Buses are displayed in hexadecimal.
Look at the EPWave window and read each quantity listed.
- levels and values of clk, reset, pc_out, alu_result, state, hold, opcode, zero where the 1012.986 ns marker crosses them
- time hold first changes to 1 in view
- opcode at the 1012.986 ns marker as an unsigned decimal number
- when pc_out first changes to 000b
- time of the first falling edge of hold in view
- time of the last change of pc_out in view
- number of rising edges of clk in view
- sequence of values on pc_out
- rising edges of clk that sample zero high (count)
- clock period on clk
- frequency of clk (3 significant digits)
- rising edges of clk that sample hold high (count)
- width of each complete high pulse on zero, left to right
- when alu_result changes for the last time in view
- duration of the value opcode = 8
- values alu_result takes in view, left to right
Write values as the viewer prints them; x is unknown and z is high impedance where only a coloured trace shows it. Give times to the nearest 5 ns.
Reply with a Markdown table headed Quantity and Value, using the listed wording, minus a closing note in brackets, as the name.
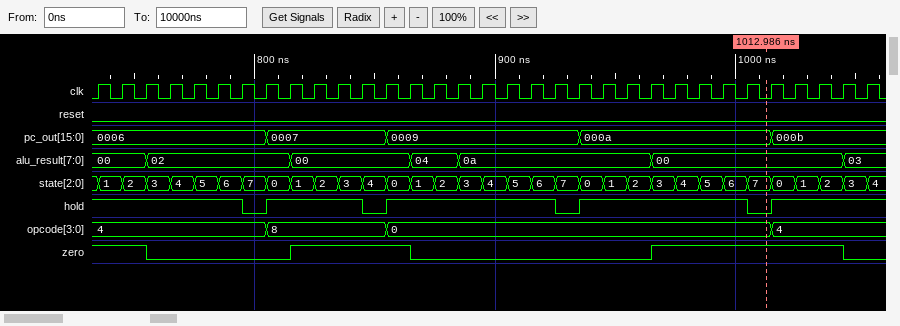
| Quantity | Value |
|---|---|
| levels and values of clk, reset, pc_out, alu_result, state, hold, opcode, zero where the 1012.986 ns marker crosses them | clk=0, reset=0, pc_out=000a, alu_result=00, state=7, hold=0, opcode=0, zero=1 |
| time hold first changes to 1 in view | 805 ns |
| opcode at the 1012.986 ns marker as an unsigned decimal number | 0 |
| when pc_out first changes to 000b | 1015 ns |
| time of the first falling edge of hold in view | 795 ns |
| time of the last change of pc_out in view | 1015 ns |
| number of rising edges of clk in view | 33 |
| sequence of values on pc_out | 0006, 0007, 0009, 000a, 000b |
| rising edges of clk that sample zero high | 16 |
| clock period on clk | 10 ns |
| frequency of clk | 100 MHz |
| rising edges of clk that sample hold high | 29 |
| width of each complete high pulse on zero, left to right | 50 ns, 80 ns |
| when alu_result changes for the last time in view | 1045 ns |
| duration of the value opcode = 8 | 50 ns |
| values alu_result takes in view, left to right | 00, 02, 00, 04, 0a, 00, 03 |
